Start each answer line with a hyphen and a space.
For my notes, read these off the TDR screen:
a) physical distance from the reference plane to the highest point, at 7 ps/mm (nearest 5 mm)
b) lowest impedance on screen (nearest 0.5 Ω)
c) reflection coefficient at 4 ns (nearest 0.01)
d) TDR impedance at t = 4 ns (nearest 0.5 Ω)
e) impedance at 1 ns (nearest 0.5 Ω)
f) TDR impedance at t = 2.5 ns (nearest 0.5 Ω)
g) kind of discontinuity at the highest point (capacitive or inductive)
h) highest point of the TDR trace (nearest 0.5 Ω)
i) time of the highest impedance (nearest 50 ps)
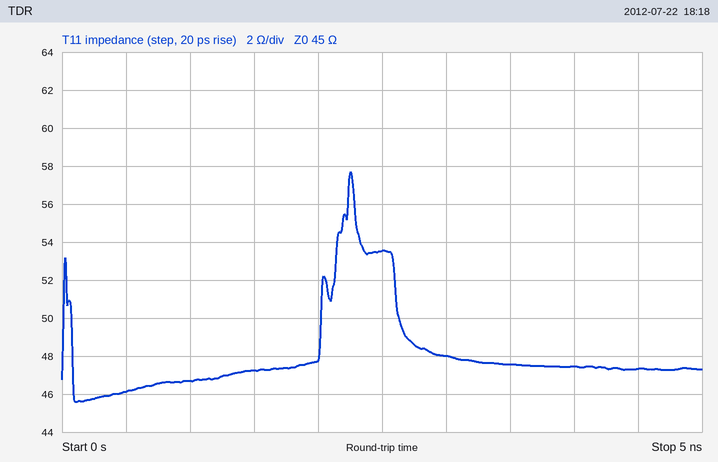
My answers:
- 160 mm
- 45.5 Ω
- +0.03
- 47.5 Ω
- 46.5 Ω
- 53.5 Ω
- inductive
- 57.5 Ω
- 2.25 ns
